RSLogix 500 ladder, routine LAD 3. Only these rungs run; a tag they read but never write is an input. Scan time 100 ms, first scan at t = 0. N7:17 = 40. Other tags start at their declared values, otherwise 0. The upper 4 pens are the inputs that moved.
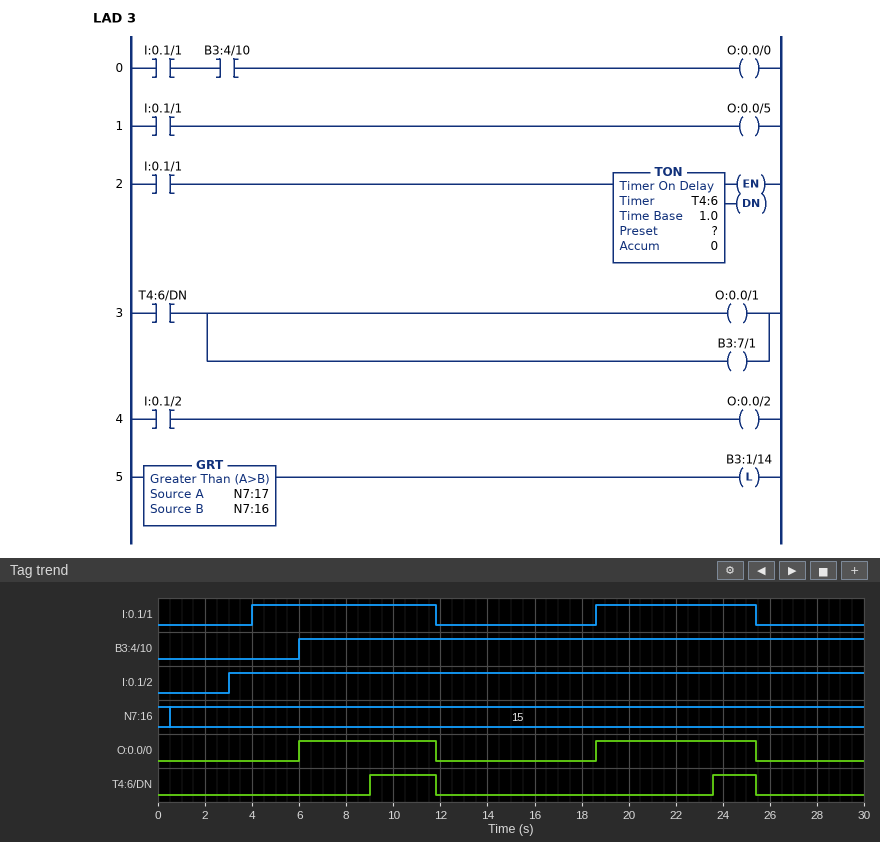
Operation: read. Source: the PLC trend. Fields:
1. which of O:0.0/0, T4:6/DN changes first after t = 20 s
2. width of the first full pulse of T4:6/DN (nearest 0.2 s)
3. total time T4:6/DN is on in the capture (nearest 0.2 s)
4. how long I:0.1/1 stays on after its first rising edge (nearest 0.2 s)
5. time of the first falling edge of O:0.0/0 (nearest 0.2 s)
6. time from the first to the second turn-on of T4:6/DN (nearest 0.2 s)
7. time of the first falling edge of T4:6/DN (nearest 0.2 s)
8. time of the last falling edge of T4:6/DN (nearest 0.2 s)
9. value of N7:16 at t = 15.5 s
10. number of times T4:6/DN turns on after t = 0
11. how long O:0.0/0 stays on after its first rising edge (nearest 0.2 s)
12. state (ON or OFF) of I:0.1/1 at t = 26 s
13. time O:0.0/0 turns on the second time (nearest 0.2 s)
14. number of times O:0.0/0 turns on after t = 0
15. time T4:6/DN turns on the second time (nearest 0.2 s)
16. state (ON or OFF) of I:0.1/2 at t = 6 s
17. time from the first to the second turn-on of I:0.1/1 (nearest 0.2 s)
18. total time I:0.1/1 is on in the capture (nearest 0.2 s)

T4:6/DN
2.8 s
4.6 s
7.8 s
11.8 s
14.6 s
11.8 s
25.4 s
15
2
5.8 s
OFF
18.6 s
2
23.6 s
ON
14.6 s
14.6 s
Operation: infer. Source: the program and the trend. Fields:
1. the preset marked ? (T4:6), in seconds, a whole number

5 s
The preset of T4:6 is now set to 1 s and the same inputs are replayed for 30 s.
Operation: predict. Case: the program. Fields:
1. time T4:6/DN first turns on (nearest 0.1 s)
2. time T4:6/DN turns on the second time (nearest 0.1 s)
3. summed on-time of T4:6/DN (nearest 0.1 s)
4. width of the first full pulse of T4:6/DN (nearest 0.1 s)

5.0 s
19.6 s
12.6 s
6.8 s
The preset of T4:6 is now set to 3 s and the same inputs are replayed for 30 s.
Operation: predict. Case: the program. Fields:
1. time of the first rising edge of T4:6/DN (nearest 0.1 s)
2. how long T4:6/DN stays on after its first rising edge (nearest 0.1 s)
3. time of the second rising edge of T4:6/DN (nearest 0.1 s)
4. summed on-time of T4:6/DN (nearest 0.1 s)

7.0 s
4.8 s
21.6 s
8.6 s
